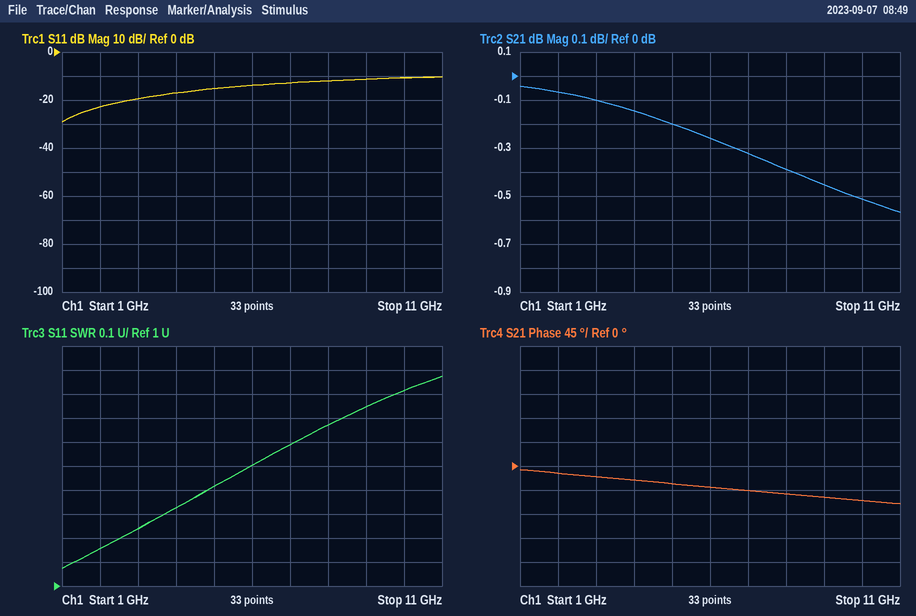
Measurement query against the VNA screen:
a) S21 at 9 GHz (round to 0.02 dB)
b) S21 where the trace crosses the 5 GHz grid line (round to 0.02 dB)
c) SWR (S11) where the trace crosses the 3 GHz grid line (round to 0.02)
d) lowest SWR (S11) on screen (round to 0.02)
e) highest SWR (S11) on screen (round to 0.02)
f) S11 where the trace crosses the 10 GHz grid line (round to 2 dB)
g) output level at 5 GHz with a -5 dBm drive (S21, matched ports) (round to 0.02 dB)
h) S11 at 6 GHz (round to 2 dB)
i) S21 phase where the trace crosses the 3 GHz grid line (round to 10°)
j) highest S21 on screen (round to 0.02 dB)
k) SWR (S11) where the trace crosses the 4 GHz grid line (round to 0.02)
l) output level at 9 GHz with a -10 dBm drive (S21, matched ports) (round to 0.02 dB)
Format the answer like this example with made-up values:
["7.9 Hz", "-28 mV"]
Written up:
["-0.46 dB", "-0.20 dB", "1.24", "1.08", "1.88", "-10 dB", "-5.20 dBm", "-14 dB", "-20°", "-0.04 dB", "1.32", "-10.46 dBm"]
